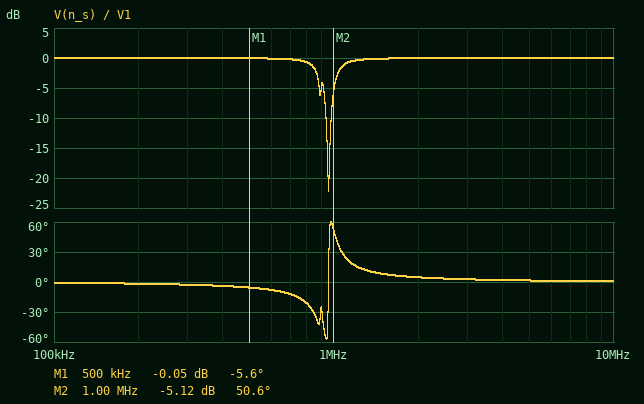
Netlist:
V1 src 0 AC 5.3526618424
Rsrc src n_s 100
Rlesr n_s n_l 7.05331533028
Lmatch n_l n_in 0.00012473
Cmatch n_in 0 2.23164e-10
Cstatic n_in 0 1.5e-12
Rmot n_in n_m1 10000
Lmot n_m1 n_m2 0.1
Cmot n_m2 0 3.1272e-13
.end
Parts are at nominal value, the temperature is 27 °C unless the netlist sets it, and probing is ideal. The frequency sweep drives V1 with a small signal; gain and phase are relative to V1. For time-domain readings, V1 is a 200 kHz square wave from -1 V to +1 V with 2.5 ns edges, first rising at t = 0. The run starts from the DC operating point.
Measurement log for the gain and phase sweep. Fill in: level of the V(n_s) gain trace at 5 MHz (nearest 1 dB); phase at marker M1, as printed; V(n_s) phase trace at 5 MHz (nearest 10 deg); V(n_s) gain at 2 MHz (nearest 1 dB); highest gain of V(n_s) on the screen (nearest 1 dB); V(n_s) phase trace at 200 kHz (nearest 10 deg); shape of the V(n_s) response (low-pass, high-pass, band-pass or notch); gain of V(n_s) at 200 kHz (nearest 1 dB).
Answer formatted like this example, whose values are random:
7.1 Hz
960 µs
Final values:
0 dB
-5.6 deg
0 deg
0 dB
0 dB
0 deg
notch
0 dB
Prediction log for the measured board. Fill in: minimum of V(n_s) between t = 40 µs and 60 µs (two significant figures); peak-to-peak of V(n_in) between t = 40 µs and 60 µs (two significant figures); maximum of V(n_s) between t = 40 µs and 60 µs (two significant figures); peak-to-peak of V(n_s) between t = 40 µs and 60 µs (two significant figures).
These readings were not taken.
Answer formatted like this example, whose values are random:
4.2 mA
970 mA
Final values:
-1.2 V
5.9 V
1.2 V
2.5 V
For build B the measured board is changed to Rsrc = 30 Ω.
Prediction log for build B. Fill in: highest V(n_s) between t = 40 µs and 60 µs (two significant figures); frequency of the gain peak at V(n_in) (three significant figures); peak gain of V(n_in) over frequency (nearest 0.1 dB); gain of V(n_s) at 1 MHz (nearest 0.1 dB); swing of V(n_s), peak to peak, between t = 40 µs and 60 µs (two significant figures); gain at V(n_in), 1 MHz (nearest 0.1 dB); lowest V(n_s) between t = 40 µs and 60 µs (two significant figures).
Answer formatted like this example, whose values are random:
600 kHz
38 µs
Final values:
1.1 V
956 kHz
25.8 dB
-1.0 dB
2.2 V
19.0 dB
-1.1 V
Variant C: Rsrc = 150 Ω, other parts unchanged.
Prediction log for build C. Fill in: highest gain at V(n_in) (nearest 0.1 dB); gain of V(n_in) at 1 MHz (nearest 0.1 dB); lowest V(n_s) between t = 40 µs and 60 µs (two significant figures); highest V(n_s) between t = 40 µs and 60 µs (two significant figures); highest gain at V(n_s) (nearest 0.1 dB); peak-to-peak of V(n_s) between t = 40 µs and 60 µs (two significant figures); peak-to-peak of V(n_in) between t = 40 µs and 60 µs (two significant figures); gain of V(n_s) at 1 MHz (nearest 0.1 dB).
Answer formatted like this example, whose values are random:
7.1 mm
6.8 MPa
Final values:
13.5 dB
12.3 dB
-1.3 V
1.3 V
0 dB
2.6 V
5.2 V
-7.7 dB
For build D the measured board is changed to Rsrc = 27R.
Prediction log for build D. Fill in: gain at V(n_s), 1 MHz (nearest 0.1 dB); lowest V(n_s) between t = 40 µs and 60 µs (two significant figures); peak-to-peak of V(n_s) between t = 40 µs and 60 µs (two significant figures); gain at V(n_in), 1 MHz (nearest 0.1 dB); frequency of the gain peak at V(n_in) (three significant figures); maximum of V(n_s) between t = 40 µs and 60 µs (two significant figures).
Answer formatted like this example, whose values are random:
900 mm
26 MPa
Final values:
-0.9 dB
-1.1 V
2.2 V
19.1 dB
956 kHz
1.1 V
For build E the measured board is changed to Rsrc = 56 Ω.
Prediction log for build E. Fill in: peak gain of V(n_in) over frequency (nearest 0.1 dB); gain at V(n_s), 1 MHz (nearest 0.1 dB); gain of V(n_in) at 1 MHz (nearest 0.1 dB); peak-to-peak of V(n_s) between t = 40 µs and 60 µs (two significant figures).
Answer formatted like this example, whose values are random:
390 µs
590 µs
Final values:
21.3 dB
-2.5 dB
17.5 dB
2.3 V
